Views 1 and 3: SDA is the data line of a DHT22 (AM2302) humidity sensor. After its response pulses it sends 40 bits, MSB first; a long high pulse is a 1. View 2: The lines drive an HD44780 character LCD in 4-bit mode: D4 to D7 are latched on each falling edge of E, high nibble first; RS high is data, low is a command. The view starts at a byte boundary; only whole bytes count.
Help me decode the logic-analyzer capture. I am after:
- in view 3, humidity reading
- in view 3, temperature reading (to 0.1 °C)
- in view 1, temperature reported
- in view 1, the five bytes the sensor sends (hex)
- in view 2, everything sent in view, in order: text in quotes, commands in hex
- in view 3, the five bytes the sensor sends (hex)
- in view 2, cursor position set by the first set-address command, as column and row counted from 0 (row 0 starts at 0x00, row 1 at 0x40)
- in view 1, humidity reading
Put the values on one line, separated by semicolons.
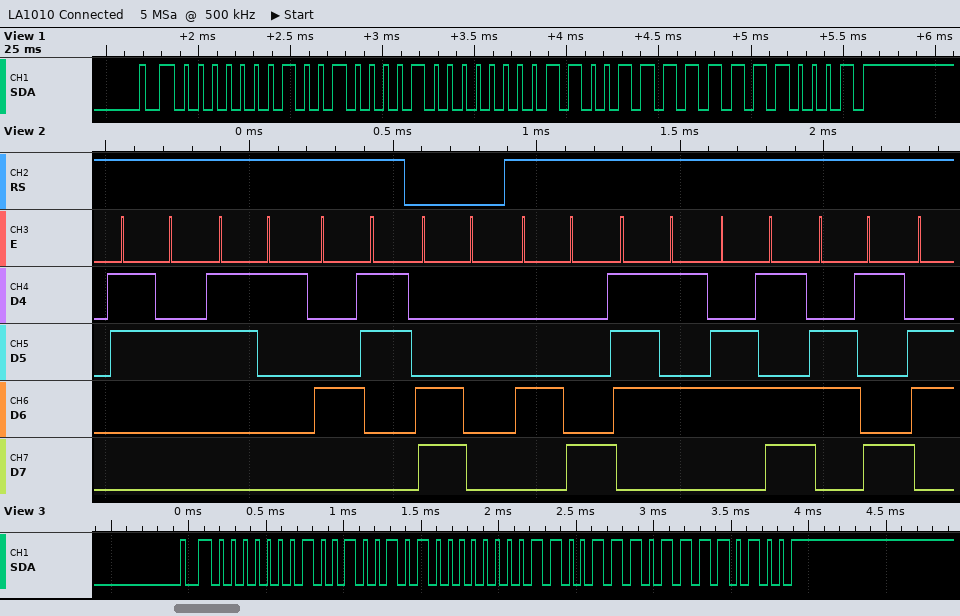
29.3 %; 20.6 °C; 20.7 °C; 01 21 00 CF F1; "21C" 0xC0 "Humi"; 01 25 00 CE F4; column 0, row 1; 28.9 %
